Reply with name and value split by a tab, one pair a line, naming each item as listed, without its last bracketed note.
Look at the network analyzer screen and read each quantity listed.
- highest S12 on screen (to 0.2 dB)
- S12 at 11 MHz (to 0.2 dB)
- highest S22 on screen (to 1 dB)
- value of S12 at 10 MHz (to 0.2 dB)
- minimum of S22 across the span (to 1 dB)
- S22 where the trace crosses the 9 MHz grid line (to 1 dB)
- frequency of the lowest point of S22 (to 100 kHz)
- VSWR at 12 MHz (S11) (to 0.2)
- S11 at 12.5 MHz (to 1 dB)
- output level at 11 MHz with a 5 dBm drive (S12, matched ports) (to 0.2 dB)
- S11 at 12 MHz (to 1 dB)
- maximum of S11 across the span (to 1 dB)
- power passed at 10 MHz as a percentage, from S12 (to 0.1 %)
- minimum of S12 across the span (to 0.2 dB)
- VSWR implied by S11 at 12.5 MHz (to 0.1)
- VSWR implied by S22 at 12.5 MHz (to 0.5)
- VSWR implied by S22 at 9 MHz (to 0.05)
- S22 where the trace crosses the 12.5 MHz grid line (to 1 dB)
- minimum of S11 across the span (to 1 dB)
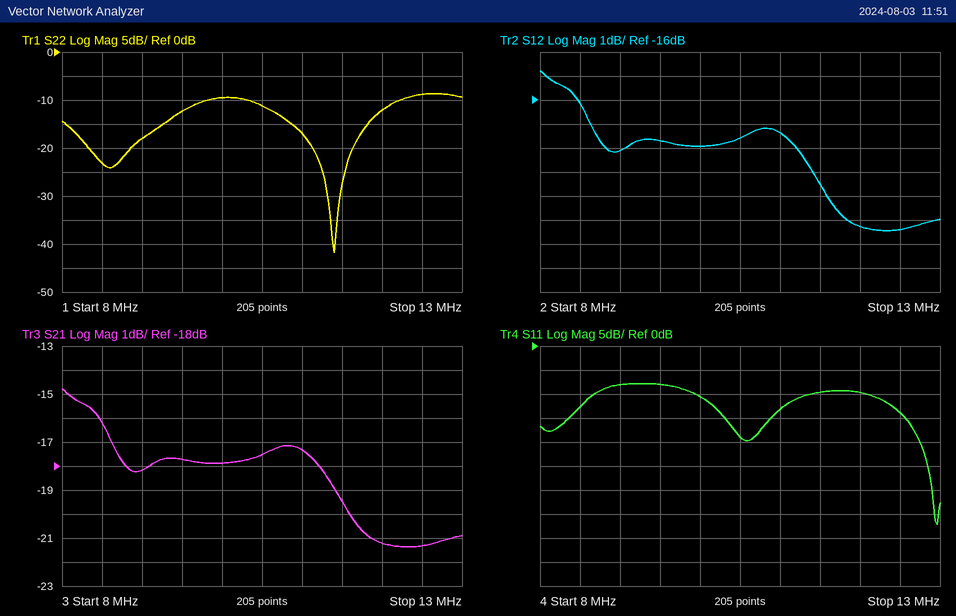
highest S12 on screen	-14.8 dB
S12 at 11 MHz	-17.4 dB
highest S22 on screen	-9 dB
value of S12 at 10 MHz	-18.0 dB
minimum of S22 across the span	-42 dB
S22 where the trace crosses the 9 MHz grid line	-18 dB
frequency of the lowest point of S22	11.4 MHz
VSWR at 12 MHz (S11)	2.0
S11 at 12.5 MHz	-14 dB
output level at 11 MHz with a 5 dBm drive (S12, matched ports)	-12.4 dBm
S11 at 12 MHz	-10 dB
maximum of S11 across the span	-8 dB
power passed at 10 MHz as a percentage, from S12	1.6 %
minimum of S12 across the span	-21.4 dB
VSWR implied by S11 at 12.5 MHz	1.5
VSWR implied by S22 at 12.5 MHz	2.0
VSWR implied by S22 at 9 MHz	1.30
S22 where the trace crosses the 12.5 MHz grid line	-9 dB
minimum of S11 across the span	-37 dB
